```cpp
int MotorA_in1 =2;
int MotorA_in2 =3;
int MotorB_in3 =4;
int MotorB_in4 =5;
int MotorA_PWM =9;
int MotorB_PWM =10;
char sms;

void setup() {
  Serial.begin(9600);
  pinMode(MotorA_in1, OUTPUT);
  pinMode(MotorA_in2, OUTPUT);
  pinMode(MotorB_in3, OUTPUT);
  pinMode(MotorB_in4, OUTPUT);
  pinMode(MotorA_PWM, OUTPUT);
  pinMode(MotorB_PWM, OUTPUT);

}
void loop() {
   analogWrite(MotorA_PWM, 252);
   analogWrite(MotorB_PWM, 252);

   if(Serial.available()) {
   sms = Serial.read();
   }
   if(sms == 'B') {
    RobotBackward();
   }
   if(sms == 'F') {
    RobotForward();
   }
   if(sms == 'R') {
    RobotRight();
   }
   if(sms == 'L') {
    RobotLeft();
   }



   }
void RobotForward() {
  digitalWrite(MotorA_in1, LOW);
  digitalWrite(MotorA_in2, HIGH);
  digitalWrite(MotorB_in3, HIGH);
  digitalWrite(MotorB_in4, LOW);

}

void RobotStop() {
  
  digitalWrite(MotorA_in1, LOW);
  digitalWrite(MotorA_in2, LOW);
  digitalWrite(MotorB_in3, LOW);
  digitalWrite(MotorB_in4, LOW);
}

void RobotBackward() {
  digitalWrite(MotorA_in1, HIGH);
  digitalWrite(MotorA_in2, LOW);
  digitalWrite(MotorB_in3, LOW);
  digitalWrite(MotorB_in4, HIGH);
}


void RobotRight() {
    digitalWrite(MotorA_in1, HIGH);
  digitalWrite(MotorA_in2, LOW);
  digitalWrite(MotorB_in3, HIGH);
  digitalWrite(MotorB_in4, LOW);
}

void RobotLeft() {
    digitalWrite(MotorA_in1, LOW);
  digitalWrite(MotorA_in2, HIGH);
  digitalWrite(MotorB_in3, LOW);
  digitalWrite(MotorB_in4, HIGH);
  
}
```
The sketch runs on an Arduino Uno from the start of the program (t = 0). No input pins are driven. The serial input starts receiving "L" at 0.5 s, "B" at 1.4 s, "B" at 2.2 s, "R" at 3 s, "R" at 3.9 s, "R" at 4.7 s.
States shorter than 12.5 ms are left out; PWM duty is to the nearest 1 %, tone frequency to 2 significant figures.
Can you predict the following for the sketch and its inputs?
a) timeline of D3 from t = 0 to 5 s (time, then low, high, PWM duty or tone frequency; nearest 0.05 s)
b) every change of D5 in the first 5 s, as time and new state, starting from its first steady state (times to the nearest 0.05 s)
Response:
0 s low; 0.5 s high; 1.4 s low
0 s low; 0.5 s high; 3 s low
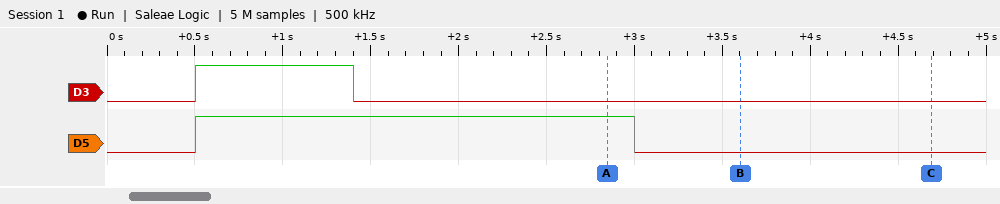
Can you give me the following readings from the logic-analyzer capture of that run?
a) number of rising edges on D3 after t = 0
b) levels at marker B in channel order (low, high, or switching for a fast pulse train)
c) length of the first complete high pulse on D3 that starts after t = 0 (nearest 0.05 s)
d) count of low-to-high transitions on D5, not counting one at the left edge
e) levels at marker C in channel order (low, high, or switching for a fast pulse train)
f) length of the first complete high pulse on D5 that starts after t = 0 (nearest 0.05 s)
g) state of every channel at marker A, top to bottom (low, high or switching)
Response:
1
D3 low, D5 low
0.90 s
1
D3 low, D5 low
2.50 s
D3 low, D5 high
